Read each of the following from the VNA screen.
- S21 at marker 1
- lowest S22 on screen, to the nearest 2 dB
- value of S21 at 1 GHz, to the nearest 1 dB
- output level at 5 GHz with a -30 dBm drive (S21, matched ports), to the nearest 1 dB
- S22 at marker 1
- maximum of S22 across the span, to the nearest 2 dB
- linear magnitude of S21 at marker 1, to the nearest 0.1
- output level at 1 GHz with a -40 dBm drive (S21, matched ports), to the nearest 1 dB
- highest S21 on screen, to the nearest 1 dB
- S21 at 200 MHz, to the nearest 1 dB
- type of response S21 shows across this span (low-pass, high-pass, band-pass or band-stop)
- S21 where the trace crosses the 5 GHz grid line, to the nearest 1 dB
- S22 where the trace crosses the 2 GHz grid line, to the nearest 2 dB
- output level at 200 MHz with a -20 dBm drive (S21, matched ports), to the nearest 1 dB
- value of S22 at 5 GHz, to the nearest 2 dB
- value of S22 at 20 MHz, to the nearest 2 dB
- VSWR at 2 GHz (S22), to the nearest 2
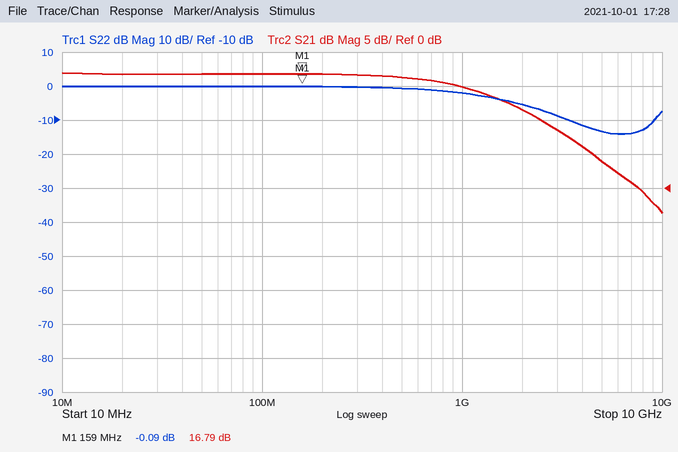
16.79 dB
-14 dB
15 dB
-26 dBm
-0.09 dB
0 dB
6.9
-25 dBm
17 dB
17 dB
low-pass
4 dB
-6 dB
-3 dBm
-14 dB
0 dB
4
